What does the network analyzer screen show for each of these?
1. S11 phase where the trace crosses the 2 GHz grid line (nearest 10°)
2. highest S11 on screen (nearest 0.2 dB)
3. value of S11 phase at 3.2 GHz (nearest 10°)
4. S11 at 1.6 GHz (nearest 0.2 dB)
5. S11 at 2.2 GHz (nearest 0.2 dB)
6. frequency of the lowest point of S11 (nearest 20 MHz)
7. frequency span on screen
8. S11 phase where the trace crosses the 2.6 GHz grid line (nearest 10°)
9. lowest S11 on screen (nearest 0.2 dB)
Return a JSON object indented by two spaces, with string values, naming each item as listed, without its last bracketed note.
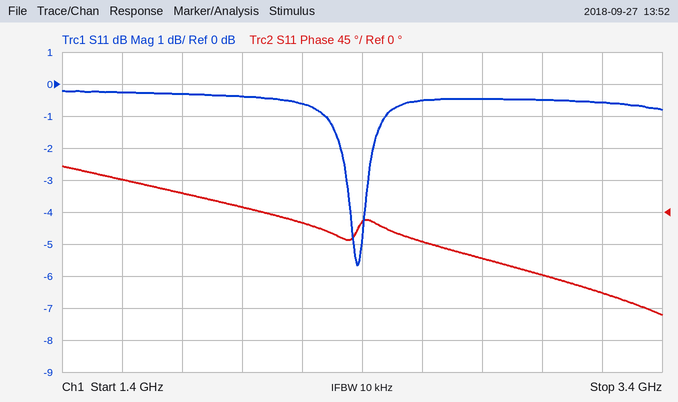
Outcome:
{
  "S11 phase where the trace crosses the 2 GHz grid line": "10°",
  "highest S11 on screen": "-0.2 dB",
  "value of S11 phase at 3.2 GHz": "-110°",
  "S11 at 1.6 GHz": "-0.2 dB",
  "S11 at 2.2 GHz": "-0.6 dB",
  "frequency of the lowest point of S11": "2.38 GHz",
  "frequency span on screen": "2 GHz",
  "S11 phase where the trace crosses the 2.6 GHz grid line": "-40°",
  "lowest S11 on screen": "-5.6 dB"
}
